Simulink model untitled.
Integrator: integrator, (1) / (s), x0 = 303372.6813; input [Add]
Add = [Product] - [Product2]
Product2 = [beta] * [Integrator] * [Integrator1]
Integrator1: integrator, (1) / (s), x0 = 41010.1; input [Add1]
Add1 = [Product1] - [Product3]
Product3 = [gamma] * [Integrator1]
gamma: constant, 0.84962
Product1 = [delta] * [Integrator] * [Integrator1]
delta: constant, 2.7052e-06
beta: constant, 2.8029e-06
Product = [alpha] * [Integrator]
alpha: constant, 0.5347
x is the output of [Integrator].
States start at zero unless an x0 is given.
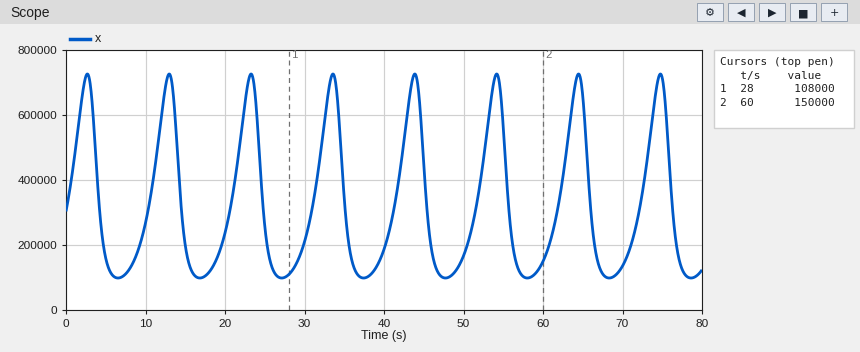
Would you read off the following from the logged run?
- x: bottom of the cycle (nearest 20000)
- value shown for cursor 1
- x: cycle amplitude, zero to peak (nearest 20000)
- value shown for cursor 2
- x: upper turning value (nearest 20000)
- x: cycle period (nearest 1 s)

100000
108000
320000
150000
720000
10 s
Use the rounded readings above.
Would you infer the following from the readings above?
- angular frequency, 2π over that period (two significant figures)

0.63 rad/s
